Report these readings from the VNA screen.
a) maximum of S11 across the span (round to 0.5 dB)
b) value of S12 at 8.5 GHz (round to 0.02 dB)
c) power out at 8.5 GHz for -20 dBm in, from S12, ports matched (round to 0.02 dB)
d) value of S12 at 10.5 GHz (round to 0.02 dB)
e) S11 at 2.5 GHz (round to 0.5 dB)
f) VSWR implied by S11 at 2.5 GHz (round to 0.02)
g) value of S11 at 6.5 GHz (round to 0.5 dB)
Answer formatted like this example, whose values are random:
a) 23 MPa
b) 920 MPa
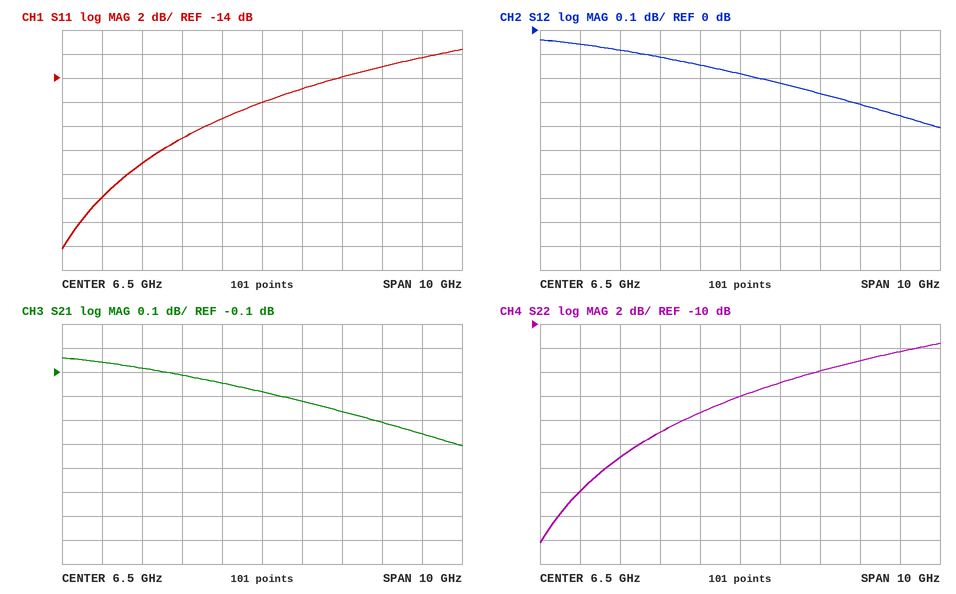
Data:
a) -11.5 dB
b) -0.26 dB
c) -20.26 dBm
d) -0.36 dB
e) -24.0 dB
f) 1.14
g) -16.0 dB
